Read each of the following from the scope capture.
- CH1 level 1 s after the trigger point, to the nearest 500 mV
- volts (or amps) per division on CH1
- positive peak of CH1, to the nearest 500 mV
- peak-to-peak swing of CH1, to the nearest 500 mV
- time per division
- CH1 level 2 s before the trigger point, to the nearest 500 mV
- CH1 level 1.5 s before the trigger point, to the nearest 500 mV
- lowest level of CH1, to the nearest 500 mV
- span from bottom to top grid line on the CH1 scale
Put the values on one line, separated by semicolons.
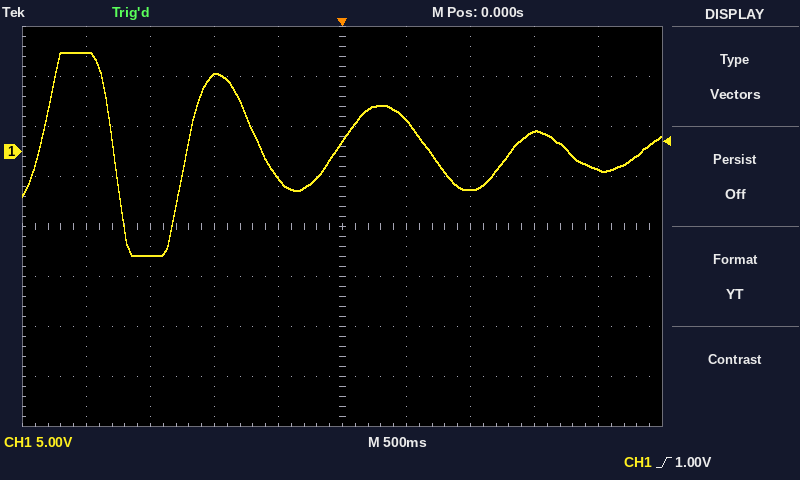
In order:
-4.0 V; 5 V; 10.0 V; 20.5 V; 500 ms; 10.0 V; -10.5 V; -10.5 V; 40 V
